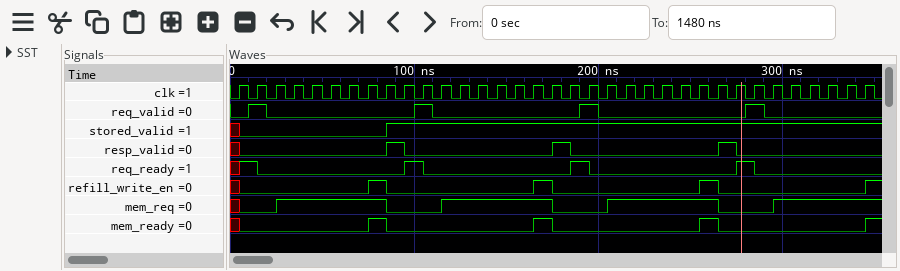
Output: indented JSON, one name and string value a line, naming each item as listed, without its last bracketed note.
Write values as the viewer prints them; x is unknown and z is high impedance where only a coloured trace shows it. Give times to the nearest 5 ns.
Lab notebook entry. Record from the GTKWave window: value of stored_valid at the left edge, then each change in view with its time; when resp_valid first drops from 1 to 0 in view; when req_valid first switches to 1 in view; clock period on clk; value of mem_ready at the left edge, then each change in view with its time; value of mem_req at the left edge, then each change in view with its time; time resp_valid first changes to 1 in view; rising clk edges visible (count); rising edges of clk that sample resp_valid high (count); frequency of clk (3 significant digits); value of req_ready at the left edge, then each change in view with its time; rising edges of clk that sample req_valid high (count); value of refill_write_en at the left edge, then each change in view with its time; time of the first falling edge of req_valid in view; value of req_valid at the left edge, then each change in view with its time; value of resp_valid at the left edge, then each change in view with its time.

{
  "value of stored_valid at the left edge, then each change in view with its time": "x, 0 at 5 ns, 1 at 85 ns",
  "when resp_valid first drops from 1 to 0 in view": "95 ns",
  "when req_valid first switches to 1 in view": "10 ns",
  "clock period on clk": "10 ns",
  "value of mem_ready at the left edge, then each change in view with its time": "x, 0 at 5 ns, 1 at 75 ns, 0 at 85 ns, 1 at 165 ns, 0 at 175 ns, 1 at 255 ns, 0 at 265 ns, 1 at 345 ns",
  "value of mem_req at the left edge, then each change in view with its time": "x, 0 at 5 ns, 1 at 25 ns, 0 at 85 ns, 1 at 115 ns, 0 at 175 ns, 1 at 205 ns, 0 at 265 ns, 1 at 295 ns",
  "time resp_valid first changes to 1 in view": "85 ns",
  "rising clk edges visible": "35",
  "rising edges of clk that sample resp_valid high": "3",
  "frequency of clk": "100 MHz",
  "value of req_ready at the left edge, then each change in view with its time": "x, 1 at 5 ns, 0 at 15 ns, 1 at 95 ns, 0 at 105 ns, 1 at 185 ns, 0 at 195 ns, 1 at 275 ns, 0 at 285 ns",
  "rising edges of clk that sample req_valid high": "4",
  "value of refill_write_en at the left edge, then each change in view with its time": "x, 0 at 5 ns, 1 at 75 ns, 0 at 85 ns, 1 at 165 ns, 0 at 175 ns, 1 at 255 ns, 0 at 265 ns, 1 at 345 ns",
  "time of the first falling edge of req_valid in view": "20 ns",
  "value of req_valid at the left edge, then each change in view with its time": "0, 1 at 10 ns, 0 at 20 ns, 1 at 100 ns, 0 at 110 ns, 1 at 190 ns, 0 at 200 ns, 1 at 280 ns, 0 at 290 ns",
  "value of resp_valid at the left edge, then each change in view with its time": "x, 0 at 5 ns, 1 at 85 ns, 0 at 95 ns, 1 at 175 ns, 0 at 185 ns, 1 at 265 ns, 0 at 275 ns"
}
